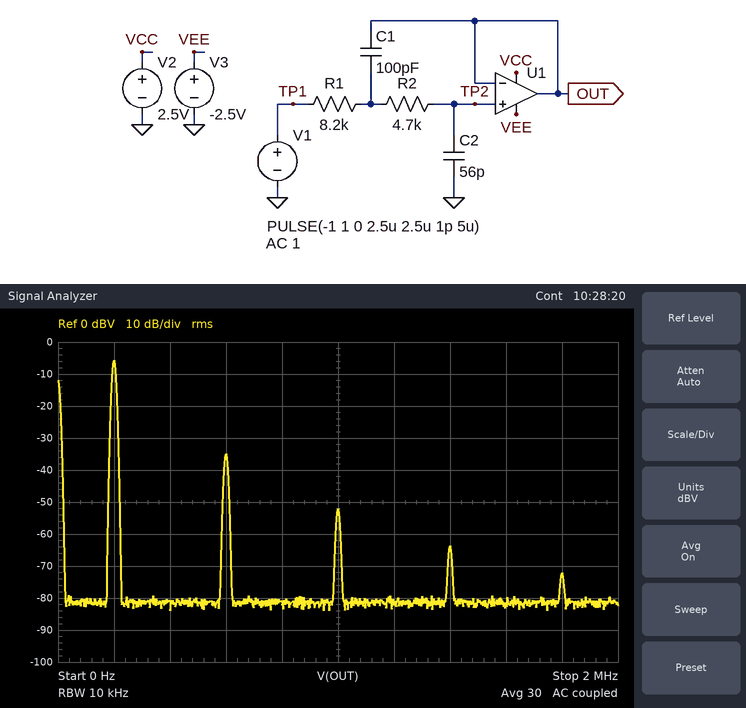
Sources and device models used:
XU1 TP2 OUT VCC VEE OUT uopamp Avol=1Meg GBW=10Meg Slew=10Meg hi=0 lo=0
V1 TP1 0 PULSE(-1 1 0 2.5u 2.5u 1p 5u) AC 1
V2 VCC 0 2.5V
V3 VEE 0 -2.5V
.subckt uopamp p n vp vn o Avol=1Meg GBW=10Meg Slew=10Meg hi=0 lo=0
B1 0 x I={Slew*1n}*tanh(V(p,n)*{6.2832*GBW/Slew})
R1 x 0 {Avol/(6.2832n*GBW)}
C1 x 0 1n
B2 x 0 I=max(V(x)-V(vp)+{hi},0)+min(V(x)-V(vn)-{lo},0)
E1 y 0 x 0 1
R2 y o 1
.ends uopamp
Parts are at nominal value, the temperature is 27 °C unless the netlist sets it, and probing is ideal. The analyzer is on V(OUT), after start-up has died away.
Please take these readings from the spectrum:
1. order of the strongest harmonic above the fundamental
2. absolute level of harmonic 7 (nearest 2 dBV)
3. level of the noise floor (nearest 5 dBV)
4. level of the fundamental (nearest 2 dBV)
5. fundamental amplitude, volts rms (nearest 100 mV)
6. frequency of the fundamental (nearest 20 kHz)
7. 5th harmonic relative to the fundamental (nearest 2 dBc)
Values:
3
-64 dBV
-80 dBV
-6 dBV
500 mV
200 kHz
-46 dBc
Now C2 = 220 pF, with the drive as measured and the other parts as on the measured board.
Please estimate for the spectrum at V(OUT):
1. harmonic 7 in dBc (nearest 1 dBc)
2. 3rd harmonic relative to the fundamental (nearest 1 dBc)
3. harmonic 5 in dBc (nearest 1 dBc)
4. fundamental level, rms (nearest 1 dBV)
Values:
-60 dBc
-32 dBc
-48 dBc
-16 dBV
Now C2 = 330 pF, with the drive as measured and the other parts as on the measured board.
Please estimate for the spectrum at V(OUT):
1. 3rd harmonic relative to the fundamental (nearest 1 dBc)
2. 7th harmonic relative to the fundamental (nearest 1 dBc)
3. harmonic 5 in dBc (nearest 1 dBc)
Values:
-32 dBc
-60 dBc
-48 dBc
